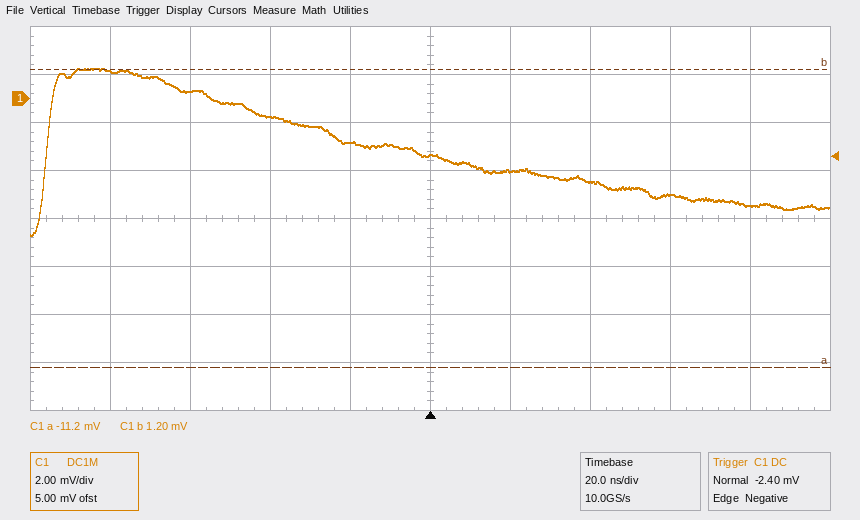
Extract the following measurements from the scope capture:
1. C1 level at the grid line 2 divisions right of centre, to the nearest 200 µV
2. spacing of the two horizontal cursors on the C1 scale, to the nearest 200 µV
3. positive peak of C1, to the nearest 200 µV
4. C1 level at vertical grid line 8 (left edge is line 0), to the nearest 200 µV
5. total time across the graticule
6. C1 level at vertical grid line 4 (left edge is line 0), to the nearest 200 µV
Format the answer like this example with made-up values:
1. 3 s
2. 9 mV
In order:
1. -3.4 mV
2. 12.4 mV
3. 1.2 mV
4. -4.0 mV
5. 200 ns
6. -1.8 mV
